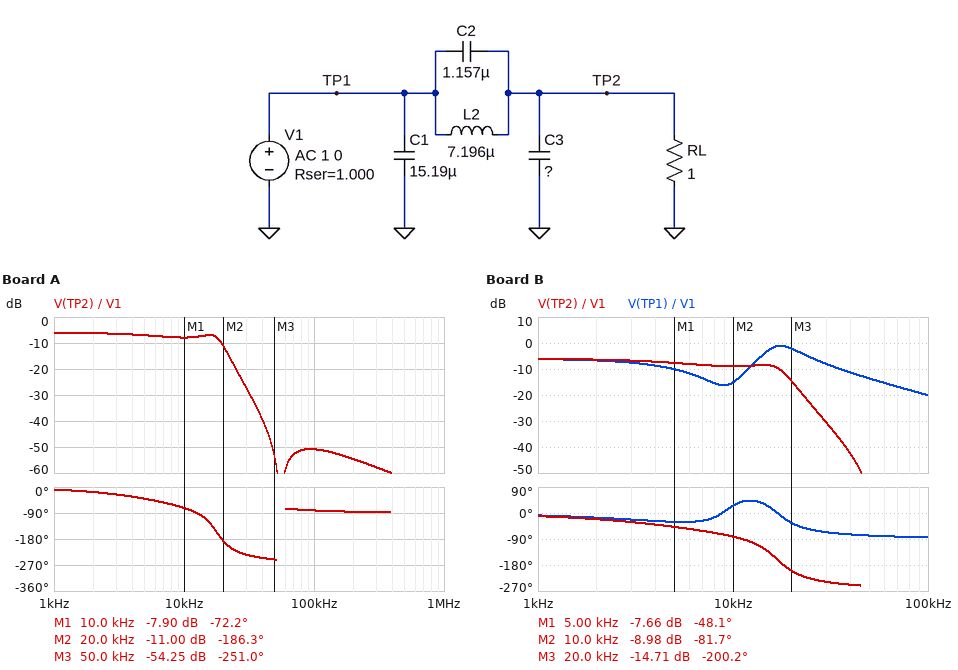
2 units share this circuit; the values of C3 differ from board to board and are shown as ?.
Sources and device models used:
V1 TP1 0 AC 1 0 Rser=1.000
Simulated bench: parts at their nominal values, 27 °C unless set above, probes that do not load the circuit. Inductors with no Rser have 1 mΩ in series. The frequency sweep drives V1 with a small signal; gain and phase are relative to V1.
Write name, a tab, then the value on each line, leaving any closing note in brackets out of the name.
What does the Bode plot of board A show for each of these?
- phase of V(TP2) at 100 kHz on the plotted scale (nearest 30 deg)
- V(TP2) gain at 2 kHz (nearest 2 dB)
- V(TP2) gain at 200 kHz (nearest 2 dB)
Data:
phase of V(TP2) at 100 kHz on the plotted scale	-90 deg
V(TP2) gain at 2 kHz	-6 dB
V(TP2) gain at 200 kHz	-54 dB
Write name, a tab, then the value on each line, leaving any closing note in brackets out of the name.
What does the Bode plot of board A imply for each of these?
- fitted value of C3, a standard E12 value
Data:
fitted value of C3, a standard E12 value	27 µF
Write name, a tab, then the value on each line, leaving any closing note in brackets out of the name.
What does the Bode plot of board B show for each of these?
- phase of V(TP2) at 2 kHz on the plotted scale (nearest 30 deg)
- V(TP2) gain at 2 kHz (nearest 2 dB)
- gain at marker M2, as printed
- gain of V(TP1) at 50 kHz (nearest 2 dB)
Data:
phase of V(TP2) at 2 kHz on the plotted scale	-30 deg
V(TP2) gain at 2 kHz	-6 dB
gain at marker M2, as printed	-8.98 dB
gain of V(TP1) at 50 kHz	-14 dB
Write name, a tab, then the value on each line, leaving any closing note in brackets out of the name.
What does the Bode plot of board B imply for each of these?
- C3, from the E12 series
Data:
C3, from the E12 series	39 µF
